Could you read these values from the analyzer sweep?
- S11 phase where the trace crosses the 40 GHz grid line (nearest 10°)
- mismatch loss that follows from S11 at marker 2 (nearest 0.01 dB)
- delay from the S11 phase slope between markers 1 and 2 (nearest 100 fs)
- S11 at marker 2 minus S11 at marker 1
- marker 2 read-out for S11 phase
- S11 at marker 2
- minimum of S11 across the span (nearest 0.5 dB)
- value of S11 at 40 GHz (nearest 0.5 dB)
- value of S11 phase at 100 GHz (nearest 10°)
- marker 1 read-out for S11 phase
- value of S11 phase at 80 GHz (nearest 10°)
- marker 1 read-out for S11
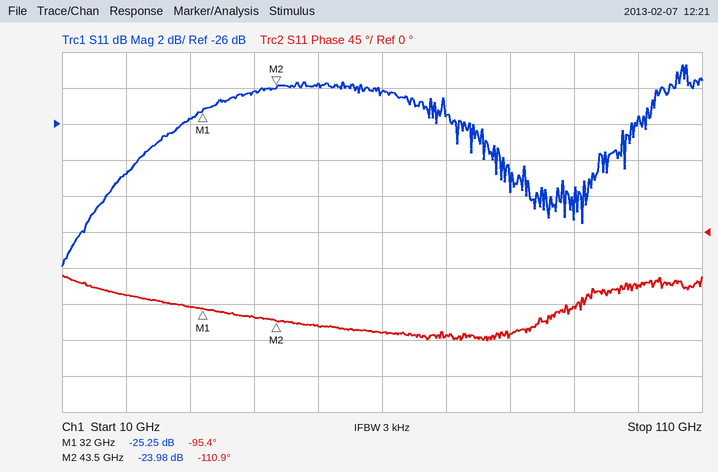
-110°
0.02 dB
3.7 ps
1.27 dB
-110.9°
-23.98 dB
-34.0 dB
-24.0 dB
-70°
-95.4°
-130°
-25.25 dB
